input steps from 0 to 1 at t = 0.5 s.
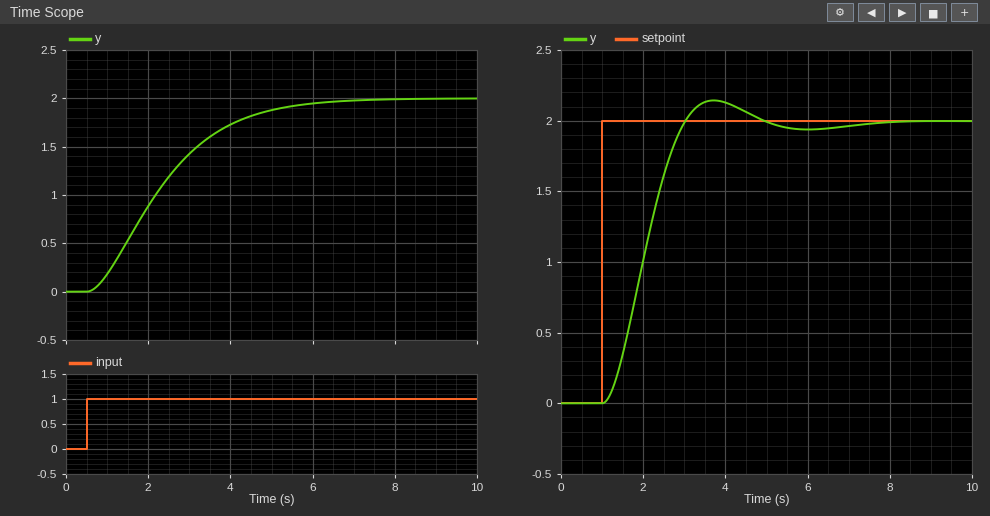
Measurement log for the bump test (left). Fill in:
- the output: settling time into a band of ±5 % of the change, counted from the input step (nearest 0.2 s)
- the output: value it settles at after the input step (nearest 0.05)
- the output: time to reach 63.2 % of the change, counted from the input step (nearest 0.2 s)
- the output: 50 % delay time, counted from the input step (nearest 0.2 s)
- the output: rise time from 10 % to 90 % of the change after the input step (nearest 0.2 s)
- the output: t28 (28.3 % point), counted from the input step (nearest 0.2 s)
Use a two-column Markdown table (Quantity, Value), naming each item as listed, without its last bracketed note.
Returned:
| Quantity | Value |
|---|---|
| the output: settling time into a band of ±5 % of the change, counted from the input step | 4.8 s |
| the output: value it settles at after the input step | 2.00 |
| the output: time to reach 63.2 % of the change, counted from the input step | 2.2 s |
| the output: 50 % delay time, counted from the input step | 1.6 s |
| the output: rise time from 10 % to 90 % of the change after the input step | 3.4 s |
| the output: t28 (28.3 % point), counted from the input step | 1.0 s |
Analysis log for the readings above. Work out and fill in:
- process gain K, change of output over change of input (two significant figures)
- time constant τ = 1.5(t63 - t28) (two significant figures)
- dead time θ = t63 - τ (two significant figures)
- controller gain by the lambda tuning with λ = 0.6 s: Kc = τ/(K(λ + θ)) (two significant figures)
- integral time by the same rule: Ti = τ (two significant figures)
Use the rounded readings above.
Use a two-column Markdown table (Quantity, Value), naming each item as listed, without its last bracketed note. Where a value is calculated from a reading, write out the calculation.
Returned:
| Quantity | Value |
|---|---|
| process gain K, change of output over change of input | (2 - 0) / 1 = 2.0 |
| time constant τ = 1.5(t63 - t28) | 1.5 × (2.2 - 1) = 1.8 s |
| dead time θ = t63 - τ | 2.2 - 1.8 = 0.40 s |
| controller gain by the lambda tuning with λ = 0.6 s: Kc = τ/(K(λ + θ)) | 1.8 / (2 × (0.6 + 0.4)) = 0.90 |
| integral time by the same rule: Ti = τ | 1.8 s |
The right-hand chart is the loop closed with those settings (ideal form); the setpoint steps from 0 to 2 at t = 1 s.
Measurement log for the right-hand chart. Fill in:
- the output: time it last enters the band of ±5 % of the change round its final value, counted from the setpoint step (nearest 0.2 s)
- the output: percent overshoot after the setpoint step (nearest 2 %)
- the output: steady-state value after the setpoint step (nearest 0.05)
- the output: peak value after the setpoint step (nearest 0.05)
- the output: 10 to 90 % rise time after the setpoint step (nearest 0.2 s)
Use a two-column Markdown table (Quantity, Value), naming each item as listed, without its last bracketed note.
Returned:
| Quantity | Value |
|---|---|
| the output: time it last enters the band of ±5 % of the change round its final value, counted from the setpoint step | 3.2 s |
| the output: percent overshoot after the setpoint step | 8 % |
| the output: steady-state value after the setpoint step | 2.00 |
| the output: peak value after the setpoint step | 2.15 |
| the output: 10 to 90 % rise time after the setpoint step | 1.4 s |
